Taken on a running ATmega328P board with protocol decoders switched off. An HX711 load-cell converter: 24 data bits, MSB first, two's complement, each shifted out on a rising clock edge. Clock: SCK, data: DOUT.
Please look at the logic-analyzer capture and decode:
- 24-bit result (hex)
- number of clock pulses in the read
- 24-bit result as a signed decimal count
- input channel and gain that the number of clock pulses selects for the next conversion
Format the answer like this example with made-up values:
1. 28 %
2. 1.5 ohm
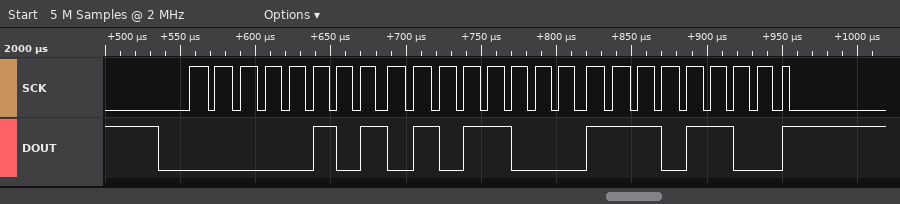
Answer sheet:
1. 0x0558EC
2. 25
3. 350444
4. channel A, gain 128
